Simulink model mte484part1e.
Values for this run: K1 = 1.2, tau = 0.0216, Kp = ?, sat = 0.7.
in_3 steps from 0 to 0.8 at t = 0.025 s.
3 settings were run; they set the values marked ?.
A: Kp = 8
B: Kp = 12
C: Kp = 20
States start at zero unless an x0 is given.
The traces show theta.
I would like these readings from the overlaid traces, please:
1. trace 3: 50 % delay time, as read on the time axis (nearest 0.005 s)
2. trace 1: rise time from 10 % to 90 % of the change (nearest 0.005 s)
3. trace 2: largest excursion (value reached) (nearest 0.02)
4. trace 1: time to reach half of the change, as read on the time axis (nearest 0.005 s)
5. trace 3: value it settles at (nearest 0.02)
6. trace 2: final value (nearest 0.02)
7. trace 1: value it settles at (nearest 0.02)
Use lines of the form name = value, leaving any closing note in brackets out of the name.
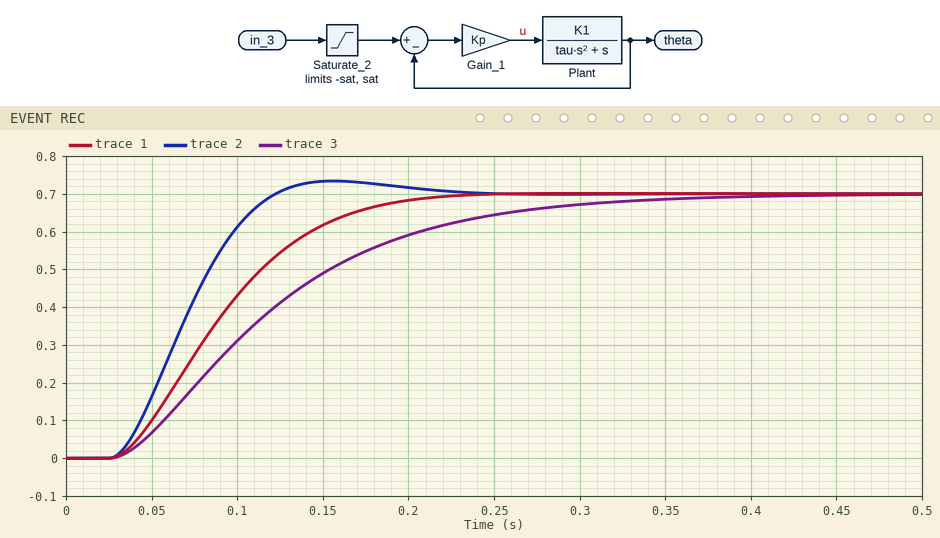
trace 3: 50 % delay time, as read on the time axis = 0.110 s
trace 1: rise time from 10 % to 90 % of the change = 0.110 s
trace 2: largest excursion (value reached) = 0.74
trace 1: time to reach half of the change, as read on the time axis = 0.085 s
trace 3: value it settles at = 0.70
trace 2: final value = 0.70
trace 1: value it settles at = 0.70
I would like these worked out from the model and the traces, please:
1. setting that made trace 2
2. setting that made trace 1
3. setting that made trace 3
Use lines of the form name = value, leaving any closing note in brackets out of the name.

setting that made trace 2 = C
setting that made trace 1 = B
setting that made trace 3 = A
